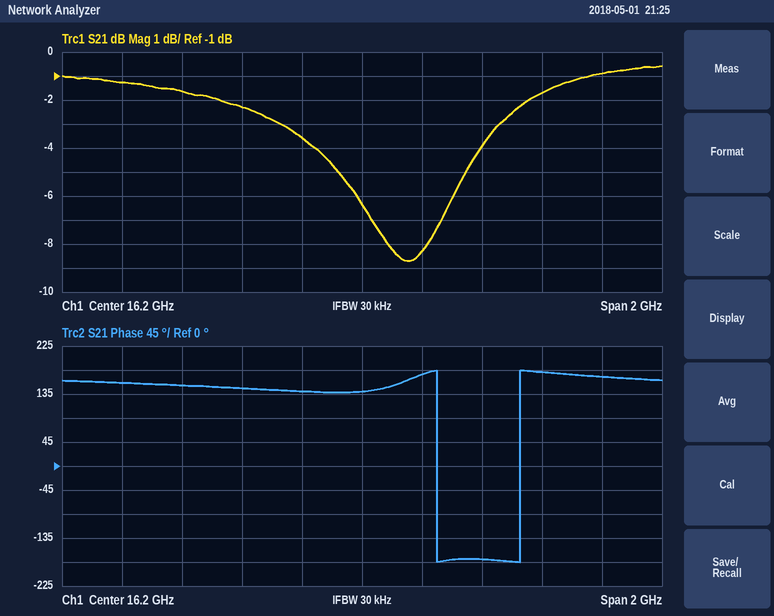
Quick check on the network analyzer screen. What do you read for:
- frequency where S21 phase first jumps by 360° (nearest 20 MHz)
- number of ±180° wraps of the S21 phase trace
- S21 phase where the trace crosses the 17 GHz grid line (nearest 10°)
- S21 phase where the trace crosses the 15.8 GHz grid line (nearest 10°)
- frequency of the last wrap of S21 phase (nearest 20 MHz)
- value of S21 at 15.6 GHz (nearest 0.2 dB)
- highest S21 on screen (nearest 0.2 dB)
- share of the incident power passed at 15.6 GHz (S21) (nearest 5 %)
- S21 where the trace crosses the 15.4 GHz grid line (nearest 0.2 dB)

16.44 GHz
2
170°
150°
16.72 GHz
-1.6 dB
-0.6 dB
70 %
-1.2 dB
